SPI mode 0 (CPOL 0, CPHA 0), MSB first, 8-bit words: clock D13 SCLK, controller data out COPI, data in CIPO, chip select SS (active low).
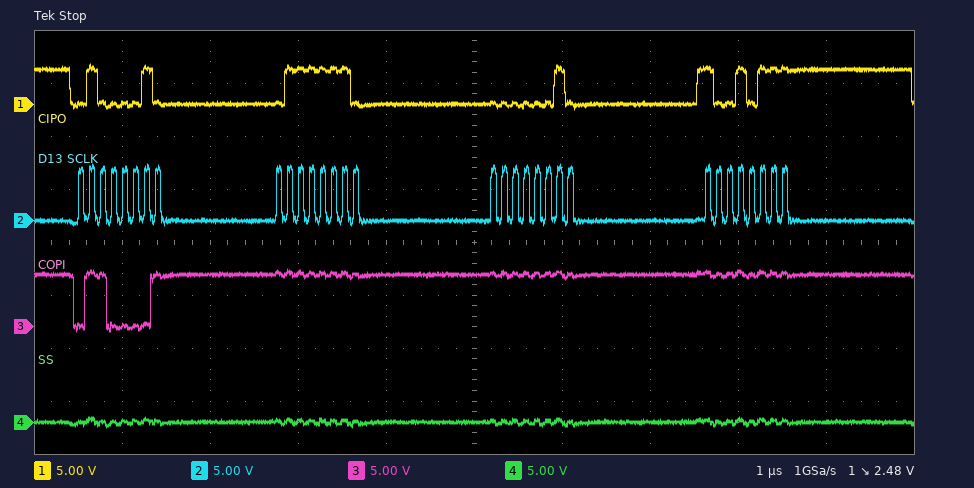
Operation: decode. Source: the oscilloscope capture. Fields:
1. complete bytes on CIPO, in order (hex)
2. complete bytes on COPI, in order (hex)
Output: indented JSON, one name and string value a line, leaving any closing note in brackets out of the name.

{
  "complete bytes on CIPO, in order": "42 7E 02 97",
  "complete bytes on COPI, in order": "61 FF FF FF"
}
